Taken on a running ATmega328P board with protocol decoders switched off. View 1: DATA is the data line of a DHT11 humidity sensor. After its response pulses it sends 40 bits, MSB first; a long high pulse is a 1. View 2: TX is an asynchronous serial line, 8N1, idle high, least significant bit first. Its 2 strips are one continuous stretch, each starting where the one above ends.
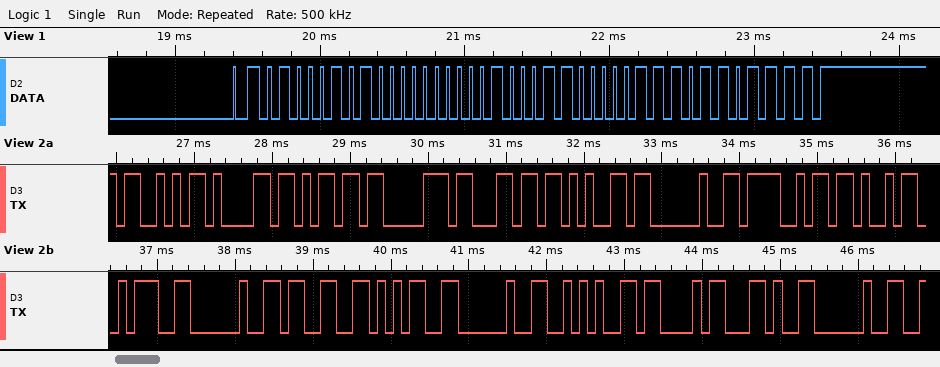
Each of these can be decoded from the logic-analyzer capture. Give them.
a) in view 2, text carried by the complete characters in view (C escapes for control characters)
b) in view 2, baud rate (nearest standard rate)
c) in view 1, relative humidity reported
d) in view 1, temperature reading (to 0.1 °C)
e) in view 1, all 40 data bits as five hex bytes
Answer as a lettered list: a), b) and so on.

a) "Sample OK: 35 *C, "
b) 9600 baud
c) 69 %
d) 35.7 °C
e) 45 00 23 07 6F
